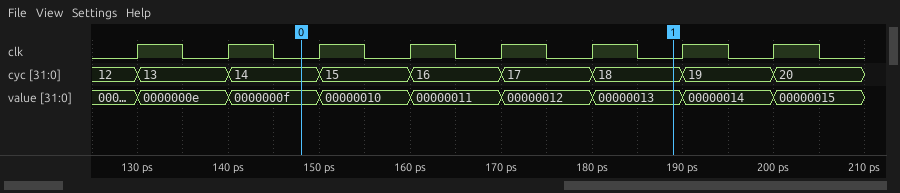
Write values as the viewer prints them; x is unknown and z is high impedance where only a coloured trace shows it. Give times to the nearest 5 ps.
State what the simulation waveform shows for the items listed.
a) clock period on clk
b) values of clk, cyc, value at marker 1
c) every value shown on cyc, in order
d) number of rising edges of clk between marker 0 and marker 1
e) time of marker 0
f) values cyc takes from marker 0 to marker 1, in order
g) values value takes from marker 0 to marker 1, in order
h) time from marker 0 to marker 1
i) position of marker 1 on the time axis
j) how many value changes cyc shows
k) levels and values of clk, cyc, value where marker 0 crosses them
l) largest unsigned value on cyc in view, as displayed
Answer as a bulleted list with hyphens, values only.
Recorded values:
- 10 ps
- clk=0, cyc=18, value=00000013
- 12, 13, 14, 15, 16, 17, 18, 19, 20
- 4
- 150 ps
- 14, 15, 16, 17, 18
- 0000000f, 00000010, 00000011, 00000012, 00000013
- 40 ps
- 190 ps
- 8
- clk=0, cyc=14, value=0000000f
- 20
